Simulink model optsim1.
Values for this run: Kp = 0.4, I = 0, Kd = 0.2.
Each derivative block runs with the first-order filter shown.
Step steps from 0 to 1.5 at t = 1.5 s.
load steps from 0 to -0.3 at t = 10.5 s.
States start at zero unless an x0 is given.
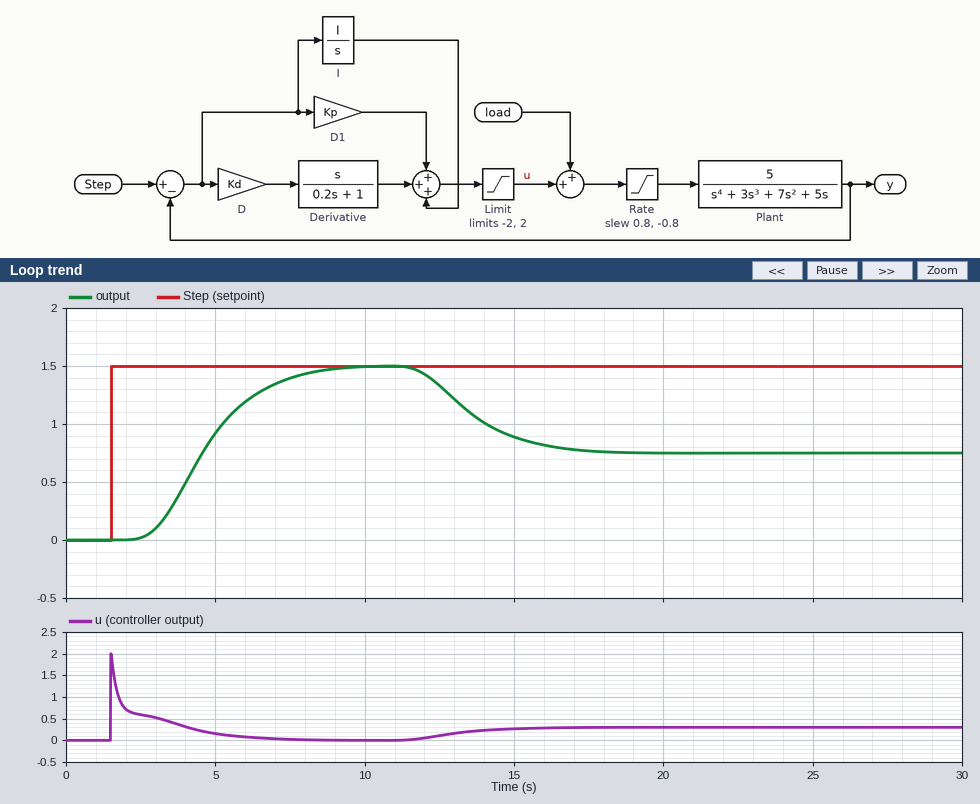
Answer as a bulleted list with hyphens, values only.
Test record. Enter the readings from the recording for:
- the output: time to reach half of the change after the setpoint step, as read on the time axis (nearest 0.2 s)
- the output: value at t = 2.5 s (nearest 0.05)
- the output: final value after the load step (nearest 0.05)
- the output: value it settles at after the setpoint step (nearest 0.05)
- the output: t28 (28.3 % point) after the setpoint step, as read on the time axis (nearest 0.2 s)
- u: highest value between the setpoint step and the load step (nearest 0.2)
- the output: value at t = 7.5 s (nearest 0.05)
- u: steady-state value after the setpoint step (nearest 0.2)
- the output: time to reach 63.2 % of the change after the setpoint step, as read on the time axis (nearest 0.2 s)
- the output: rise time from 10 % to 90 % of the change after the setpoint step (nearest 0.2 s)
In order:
- 4.6 s
- 0.00
- 0.75
- 1.50
- 3.8 s
- 2.0
- 1.40
- 0.0
- 5.0 s
- 3.8 s
